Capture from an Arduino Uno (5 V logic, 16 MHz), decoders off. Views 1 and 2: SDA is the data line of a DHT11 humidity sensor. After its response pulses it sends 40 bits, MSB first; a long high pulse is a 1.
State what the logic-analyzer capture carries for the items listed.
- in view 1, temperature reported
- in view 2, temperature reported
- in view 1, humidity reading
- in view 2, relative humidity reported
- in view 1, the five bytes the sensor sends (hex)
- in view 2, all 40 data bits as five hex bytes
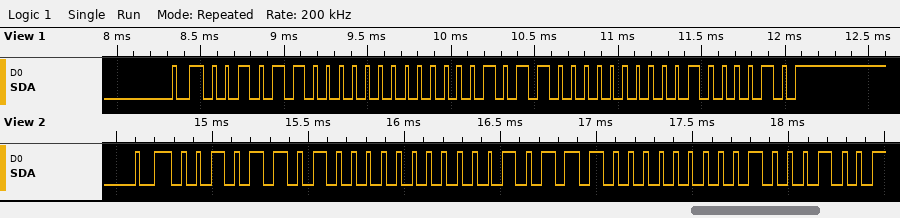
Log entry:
22.0 °C
23.0 °C
44 %
45 %
2C 00 16 00 42
2D 00 17 00 44
